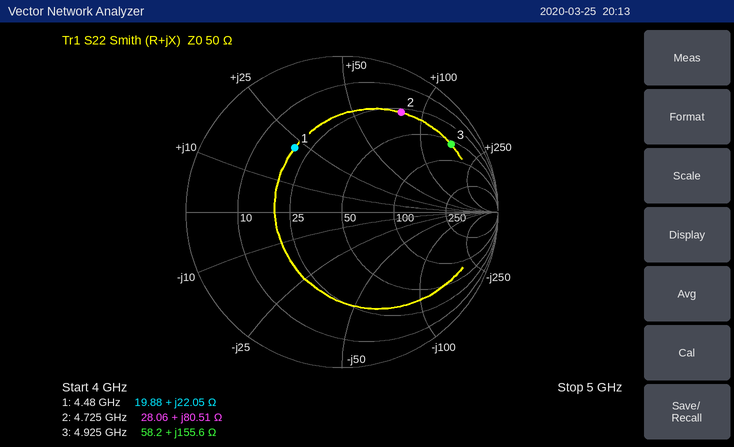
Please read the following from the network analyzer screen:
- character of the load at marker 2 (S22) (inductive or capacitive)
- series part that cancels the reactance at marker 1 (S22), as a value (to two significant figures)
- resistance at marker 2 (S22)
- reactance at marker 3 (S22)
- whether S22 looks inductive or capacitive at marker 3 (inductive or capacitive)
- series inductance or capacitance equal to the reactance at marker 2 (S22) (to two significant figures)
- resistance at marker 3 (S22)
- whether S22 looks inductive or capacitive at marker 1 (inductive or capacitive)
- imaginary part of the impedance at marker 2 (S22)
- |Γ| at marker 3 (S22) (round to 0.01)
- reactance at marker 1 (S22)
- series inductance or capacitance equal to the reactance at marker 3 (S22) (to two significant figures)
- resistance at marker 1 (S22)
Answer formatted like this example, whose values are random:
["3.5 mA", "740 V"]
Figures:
["inductive", "1.6 pF", "28.06 Ω", "+155.6 Ω", "inductive", "2.7 nH", "58.2 Ω", "inductive", "+80.51 Ω", "0.82", "+22.05 Ω", "5.0 nH", "19.88 Ω"]
